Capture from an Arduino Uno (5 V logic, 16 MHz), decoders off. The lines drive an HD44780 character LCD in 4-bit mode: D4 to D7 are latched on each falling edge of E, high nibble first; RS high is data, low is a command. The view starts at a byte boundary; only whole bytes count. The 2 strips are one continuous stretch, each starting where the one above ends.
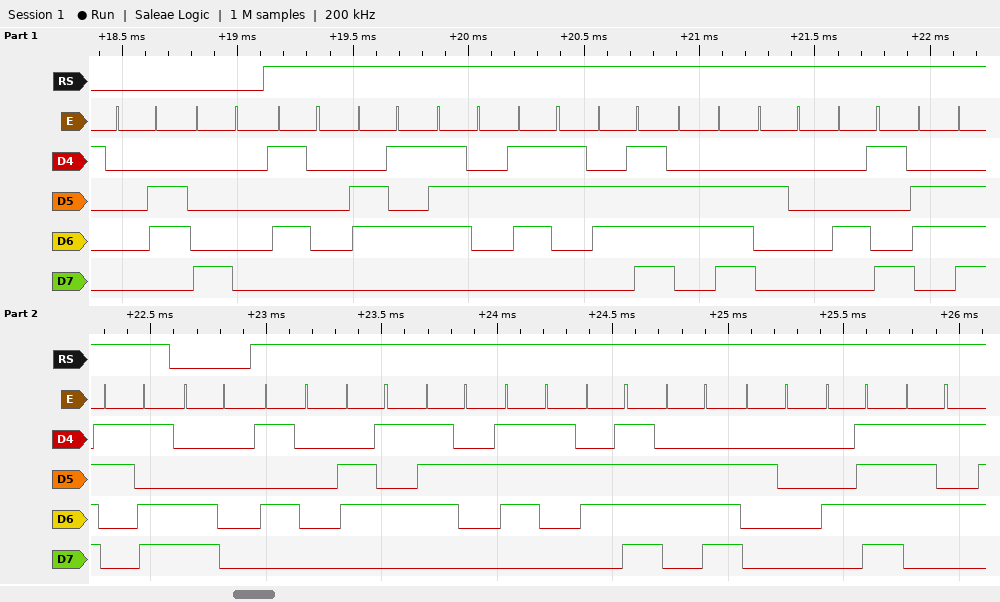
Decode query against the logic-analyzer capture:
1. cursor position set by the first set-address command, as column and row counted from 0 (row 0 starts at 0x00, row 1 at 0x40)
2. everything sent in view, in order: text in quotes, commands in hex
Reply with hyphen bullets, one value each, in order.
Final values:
- column 0, row 0
- 0x06 0x80 "Person In=" 0xC0 "Person Ou"
